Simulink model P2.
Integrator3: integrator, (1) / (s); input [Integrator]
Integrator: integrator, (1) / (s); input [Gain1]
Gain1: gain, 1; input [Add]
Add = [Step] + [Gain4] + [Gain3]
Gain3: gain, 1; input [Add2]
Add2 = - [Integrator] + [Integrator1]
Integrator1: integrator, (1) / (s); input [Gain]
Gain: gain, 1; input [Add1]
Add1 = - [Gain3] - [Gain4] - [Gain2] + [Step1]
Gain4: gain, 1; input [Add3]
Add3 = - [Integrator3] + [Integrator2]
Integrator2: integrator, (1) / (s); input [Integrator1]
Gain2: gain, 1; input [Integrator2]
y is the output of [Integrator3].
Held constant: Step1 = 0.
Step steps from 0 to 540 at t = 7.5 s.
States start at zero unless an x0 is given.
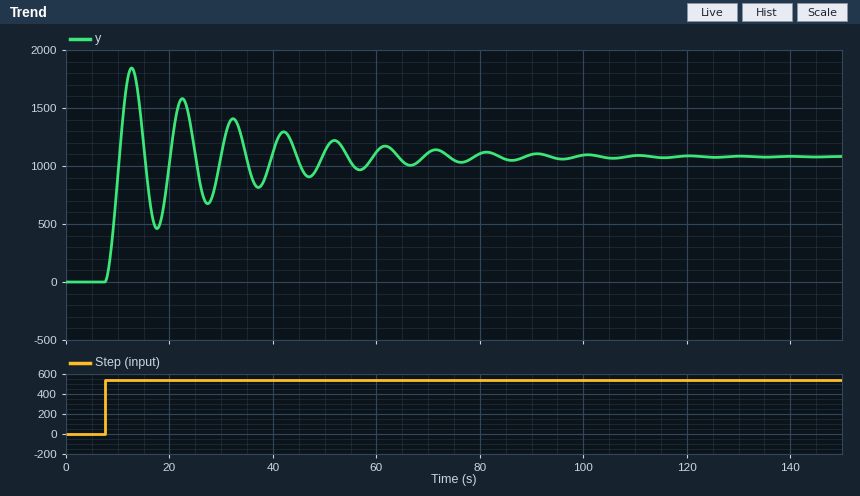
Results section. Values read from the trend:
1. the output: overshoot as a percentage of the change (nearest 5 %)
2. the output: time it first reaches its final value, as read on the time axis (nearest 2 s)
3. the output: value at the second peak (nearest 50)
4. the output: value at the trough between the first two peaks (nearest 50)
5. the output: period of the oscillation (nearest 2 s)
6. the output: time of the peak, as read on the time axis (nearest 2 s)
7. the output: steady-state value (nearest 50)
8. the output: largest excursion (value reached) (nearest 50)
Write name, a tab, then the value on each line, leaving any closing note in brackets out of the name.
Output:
the output: overshoot as a percentage of the change	70 %
the output: time it first reaches its final value, as read on the time axis	10 s
the output: value at the second peak	1600
the output: value at the trough between the first two peaks	450
the output: period of the oscillation	10 s
the output: time of the peak, as read on the time axis	12 s
the output: steady-state value	1100
the output: largest excursion (value reached)	1850
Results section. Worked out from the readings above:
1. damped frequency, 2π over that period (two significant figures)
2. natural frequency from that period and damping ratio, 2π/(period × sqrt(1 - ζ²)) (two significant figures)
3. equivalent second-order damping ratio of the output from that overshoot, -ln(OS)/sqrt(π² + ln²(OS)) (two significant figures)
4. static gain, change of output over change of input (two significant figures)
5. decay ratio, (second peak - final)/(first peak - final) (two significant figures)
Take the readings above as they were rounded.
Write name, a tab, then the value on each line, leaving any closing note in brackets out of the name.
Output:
damped frequency, 2π over that period	0.63 rad/s
natural frequency from that period and damping ratio, 2π/(period × sqrt(1 - ζ²))	0.63 rad/s
equivalent second-order damping ratio of the output from that overshoot, -ln(OS)/sqrt(π² + ln²(OS))	0.11
static gain, change of output over change of input	2.0
decay ratio, (second peak - final)/(first peak - final)	0.67
